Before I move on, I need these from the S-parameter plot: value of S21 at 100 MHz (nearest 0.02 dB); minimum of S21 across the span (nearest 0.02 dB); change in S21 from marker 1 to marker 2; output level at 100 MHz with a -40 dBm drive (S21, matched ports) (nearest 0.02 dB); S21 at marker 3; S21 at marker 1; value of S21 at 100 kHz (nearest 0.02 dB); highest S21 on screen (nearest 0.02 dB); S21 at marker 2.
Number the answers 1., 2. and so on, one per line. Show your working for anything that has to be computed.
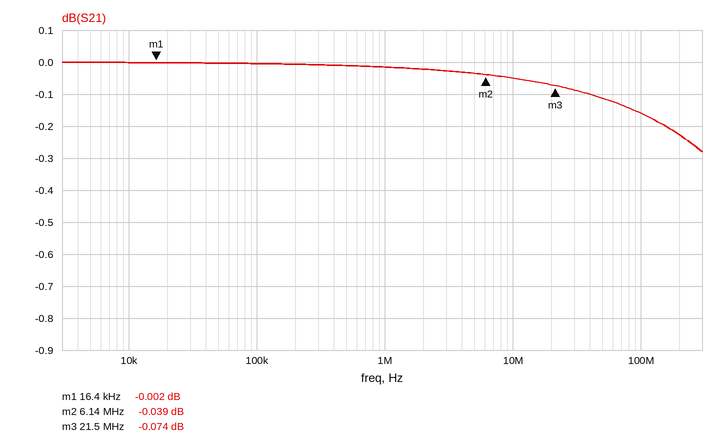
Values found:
1. -0.16 dB
2. -0.28 dB
3. -0.039 − (-0.002) = -0.037 dB
4. -40 dBm + (-0.16 dB) = -40.16 dBm
5. -0.074 dB
6. -0.002 dB
7. 0.00 dB
8. 0.00 dB
9. -0.039 dB
